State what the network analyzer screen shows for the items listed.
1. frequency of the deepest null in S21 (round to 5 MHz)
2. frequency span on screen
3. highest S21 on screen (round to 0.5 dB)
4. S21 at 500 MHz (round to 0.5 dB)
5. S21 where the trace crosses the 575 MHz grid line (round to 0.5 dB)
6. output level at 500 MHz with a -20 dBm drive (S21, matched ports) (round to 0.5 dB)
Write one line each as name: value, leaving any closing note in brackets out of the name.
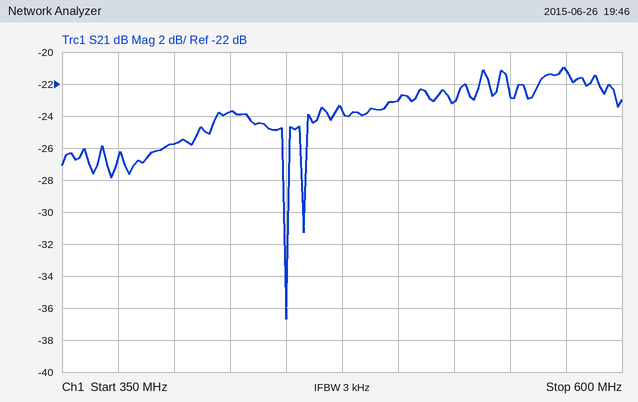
frequency of the deepest null in S21: 450 MHz
frequency span on screen: 250 MHz
highest S21 on screen: -21.0 dB
S21 at 500 MHz: -23.0 dB
S21 where the trace crosses the 575 MHz grid line: -21.0 dB
output level at 500 MHz with a -20 dBm drive (S21, matched ports): -43.0 dBm
